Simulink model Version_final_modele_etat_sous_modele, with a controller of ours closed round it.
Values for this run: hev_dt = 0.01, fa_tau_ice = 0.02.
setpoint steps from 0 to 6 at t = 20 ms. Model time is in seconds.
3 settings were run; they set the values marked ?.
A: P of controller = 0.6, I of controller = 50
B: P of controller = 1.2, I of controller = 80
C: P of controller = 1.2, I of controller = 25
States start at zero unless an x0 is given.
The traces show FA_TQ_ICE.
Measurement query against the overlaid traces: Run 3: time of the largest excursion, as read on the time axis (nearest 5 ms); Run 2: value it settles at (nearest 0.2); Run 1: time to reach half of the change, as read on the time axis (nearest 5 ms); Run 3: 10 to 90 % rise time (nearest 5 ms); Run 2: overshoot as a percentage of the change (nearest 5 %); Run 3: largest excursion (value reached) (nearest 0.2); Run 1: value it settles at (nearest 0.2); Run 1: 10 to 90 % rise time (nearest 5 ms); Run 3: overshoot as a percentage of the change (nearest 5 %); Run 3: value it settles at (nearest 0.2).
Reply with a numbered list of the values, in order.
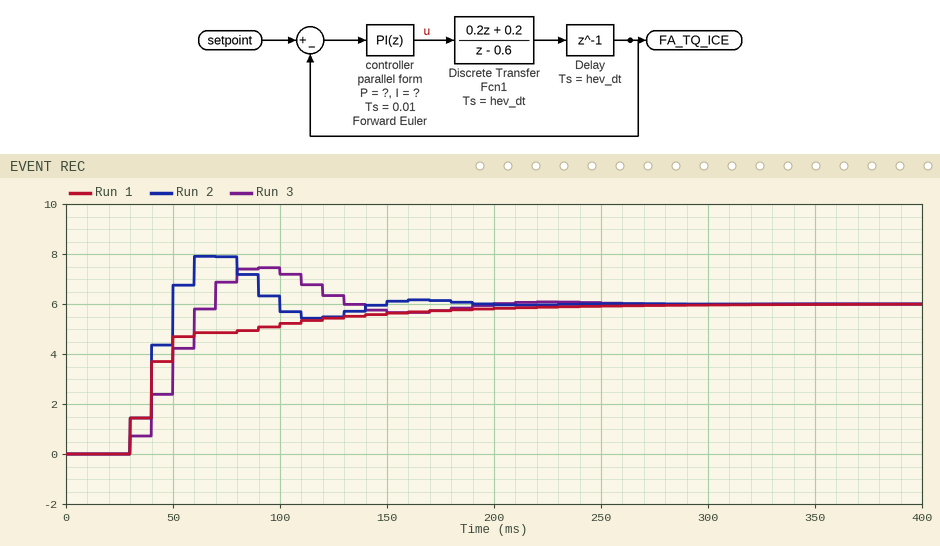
1. 90 ms
2. 6.0
3. 40 ms
4. 30 ms
5. 30 %
6. 7.4
7. 6.0
8. 90 ms
9. 25 %
10. 6.0
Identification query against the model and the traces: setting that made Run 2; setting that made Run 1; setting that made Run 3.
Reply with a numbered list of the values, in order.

1. B
2. C
3. A
